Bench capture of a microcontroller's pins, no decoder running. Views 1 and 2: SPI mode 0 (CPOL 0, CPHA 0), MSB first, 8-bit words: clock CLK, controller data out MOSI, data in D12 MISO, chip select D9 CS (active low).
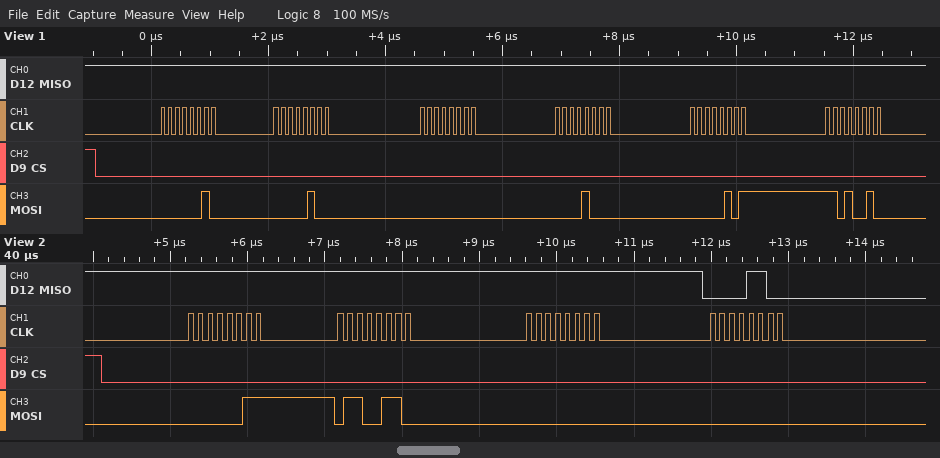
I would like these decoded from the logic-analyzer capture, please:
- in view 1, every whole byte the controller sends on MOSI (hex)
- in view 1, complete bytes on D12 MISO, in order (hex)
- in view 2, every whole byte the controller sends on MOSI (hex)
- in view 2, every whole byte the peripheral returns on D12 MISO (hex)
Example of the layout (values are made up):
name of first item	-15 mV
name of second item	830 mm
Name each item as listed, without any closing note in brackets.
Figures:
in view 1, every whole byte the controller sends on MOSI	0x02 0x04 0x00 0x08 0x05 0xD2
in view 1, complete bytes on D12 MISO, in order	0xFF 0xFF 0xFF 0xFF 0xFF 0xFF
in view 2, every whole byte the controller sends on MOSI	0x03 0x66 0x00 0x00
in view 2, every whole byte the peripheral returns on D12 MISO	0xFF 0xFF 0xFF 0x0C
